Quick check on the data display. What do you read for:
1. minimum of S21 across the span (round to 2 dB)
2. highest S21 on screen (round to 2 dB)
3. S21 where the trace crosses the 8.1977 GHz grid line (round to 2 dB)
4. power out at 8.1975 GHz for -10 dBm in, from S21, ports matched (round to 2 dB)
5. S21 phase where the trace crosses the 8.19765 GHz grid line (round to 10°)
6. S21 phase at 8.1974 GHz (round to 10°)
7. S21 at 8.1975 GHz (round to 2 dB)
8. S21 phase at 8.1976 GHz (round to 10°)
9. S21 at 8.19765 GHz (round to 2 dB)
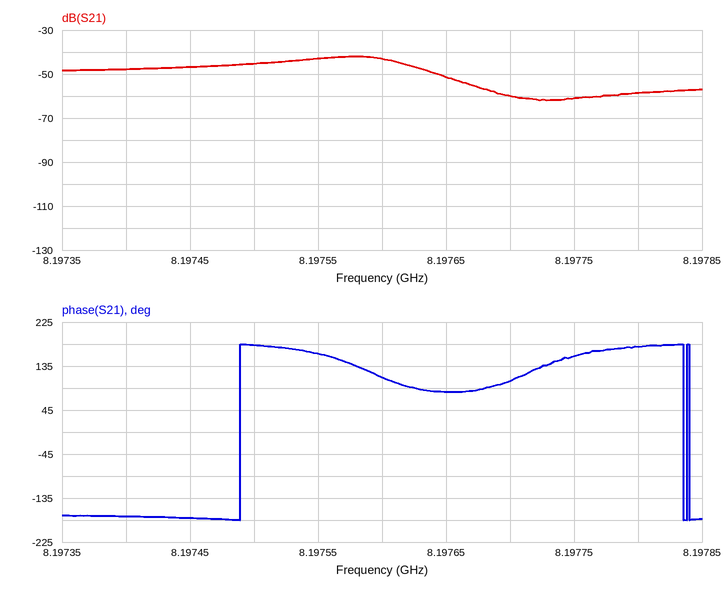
-62 dB
-42 dB
-60 dB
-56 dBm
80°
-170°
-46 dB
110°
-52 dB
